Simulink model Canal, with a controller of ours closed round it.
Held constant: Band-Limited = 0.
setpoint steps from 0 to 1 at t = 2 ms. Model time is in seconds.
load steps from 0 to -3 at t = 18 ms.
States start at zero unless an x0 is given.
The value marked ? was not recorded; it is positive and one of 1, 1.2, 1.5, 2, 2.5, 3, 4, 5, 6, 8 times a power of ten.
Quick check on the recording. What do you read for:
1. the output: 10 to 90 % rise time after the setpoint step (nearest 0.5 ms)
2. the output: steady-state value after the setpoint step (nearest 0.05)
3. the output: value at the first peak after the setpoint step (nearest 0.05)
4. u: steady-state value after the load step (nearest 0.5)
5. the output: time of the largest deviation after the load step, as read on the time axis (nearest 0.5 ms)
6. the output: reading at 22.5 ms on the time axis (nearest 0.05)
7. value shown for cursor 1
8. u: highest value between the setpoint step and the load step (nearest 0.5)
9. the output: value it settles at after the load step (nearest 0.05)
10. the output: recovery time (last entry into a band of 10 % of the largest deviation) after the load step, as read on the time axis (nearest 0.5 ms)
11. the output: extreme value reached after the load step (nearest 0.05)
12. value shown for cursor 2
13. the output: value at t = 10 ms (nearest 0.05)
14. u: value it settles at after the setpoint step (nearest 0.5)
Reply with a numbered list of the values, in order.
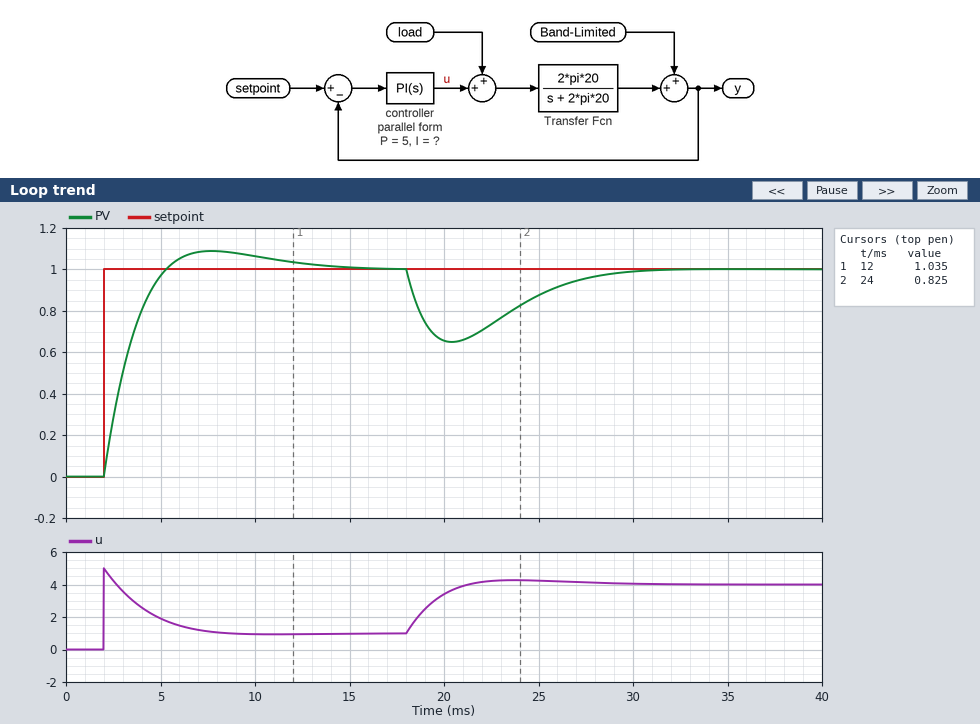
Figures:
1. 2.5 ms
2. 1.00
3. 1.10
4. 4.0
5. 20.5 ms
6. 0.75
7. 1.035
8. 5.0
9. 1.00
10. 28.0 ms
11. 0.65
12. 0.825
13. 1.05
14. 1.0
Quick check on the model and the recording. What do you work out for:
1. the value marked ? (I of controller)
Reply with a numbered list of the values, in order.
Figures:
1. 1500
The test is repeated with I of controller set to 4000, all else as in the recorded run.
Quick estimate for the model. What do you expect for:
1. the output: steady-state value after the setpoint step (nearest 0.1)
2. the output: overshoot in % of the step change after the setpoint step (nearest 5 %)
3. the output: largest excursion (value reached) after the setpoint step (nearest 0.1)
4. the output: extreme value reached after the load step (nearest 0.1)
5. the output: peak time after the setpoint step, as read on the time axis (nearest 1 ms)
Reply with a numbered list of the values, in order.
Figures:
1. 1.0
2. 25 %
3. 1.2
4. 0.7
5. 6 ms
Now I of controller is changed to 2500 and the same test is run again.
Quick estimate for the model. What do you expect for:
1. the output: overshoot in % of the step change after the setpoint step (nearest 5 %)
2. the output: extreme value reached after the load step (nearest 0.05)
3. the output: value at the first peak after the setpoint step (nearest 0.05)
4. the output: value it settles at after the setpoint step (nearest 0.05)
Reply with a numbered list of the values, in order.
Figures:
1. 15 %
2. 0.70
3. 1.15
4. 1.00
